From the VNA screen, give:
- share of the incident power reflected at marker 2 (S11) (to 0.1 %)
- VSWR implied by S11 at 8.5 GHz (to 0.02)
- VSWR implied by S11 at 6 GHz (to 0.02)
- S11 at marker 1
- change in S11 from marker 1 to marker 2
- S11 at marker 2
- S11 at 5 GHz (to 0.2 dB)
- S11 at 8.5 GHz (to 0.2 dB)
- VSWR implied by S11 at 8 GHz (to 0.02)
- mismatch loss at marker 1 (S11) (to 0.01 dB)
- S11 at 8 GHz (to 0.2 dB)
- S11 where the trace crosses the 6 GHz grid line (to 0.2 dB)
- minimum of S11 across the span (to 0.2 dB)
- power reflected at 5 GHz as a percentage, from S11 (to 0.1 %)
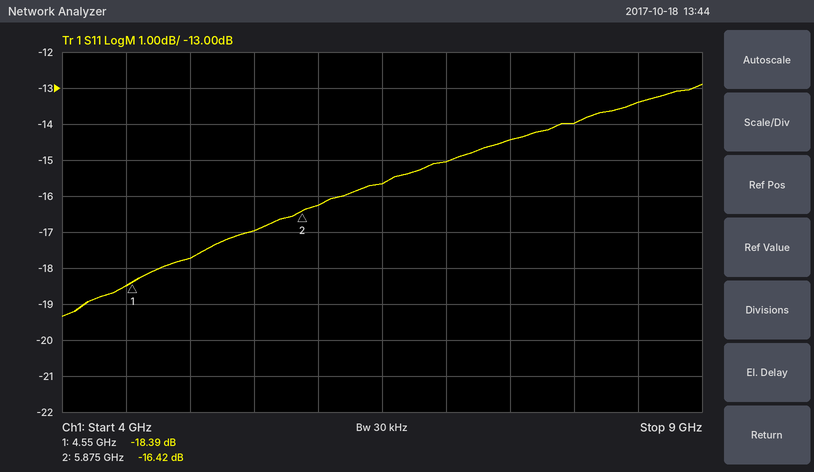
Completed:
2.3 %
1.54
1.36
-18.39 dB
1.97 dB
-16.42 dB
-17.8 dB
-13.4 dB
1.50
0.06 dB
-14.0 dB
-16.2 dB
-19.4 dB
1.7 %
